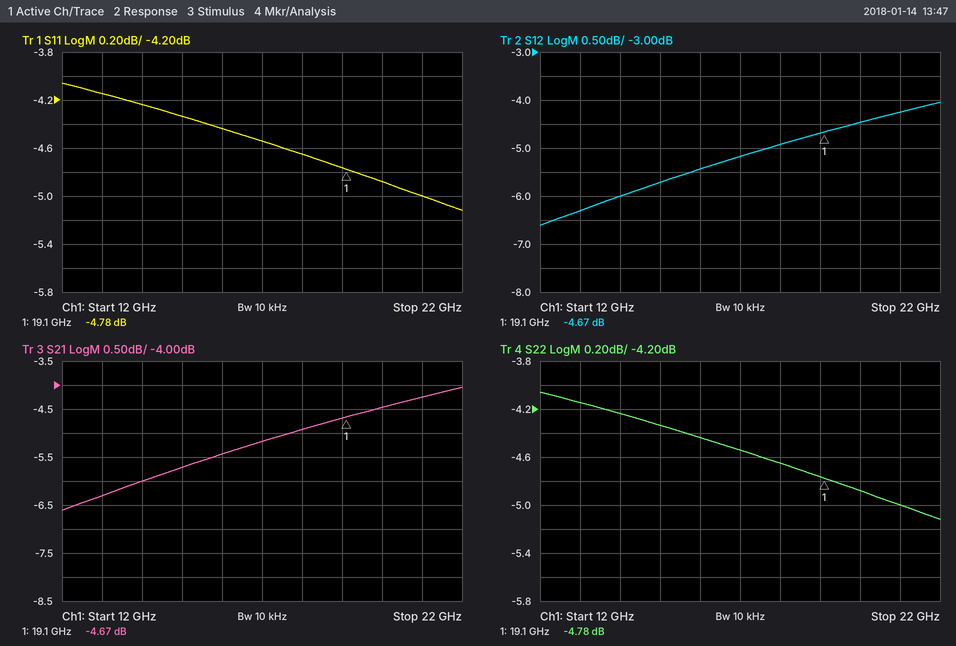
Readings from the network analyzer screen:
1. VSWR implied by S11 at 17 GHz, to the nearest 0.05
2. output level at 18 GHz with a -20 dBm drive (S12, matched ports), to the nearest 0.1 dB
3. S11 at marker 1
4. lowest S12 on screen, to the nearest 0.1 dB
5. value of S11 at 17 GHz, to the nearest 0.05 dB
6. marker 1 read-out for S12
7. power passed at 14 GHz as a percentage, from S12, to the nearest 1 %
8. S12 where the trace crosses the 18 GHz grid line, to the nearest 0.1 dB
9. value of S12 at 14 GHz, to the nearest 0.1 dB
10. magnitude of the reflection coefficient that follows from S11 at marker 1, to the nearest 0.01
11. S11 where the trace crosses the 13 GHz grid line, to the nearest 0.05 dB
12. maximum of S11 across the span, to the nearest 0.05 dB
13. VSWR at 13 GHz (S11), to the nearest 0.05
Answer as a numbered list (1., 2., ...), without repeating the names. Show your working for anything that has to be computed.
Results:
1. |Γ| = 10^(-4.55/20) = 0.5922; VSWR = (1 + 0.5922)/(1 − 0.5922) ≈ 3.90
2. -20 dBm + (-4.9 dB) = -24.9 dBm
3. -4.78 dB
4. -6.6 dB
5. -4.55 dB
6. -4.67 dB
7. 10^(-6/10) ≈ 25 %
8. -4.9 dB
9. -6.0 dB
10. 10^(-4.78/20) ≈ 0.58
11. -4.15 dB
12. -4.05 dB
13. |Γ| = 10^(-4.15/20) = 0.6202; VSWR = (1 + 0.6202)/(1 − 0.6202) ≈ 4.27, so 4.25 to the nearest 0.05
